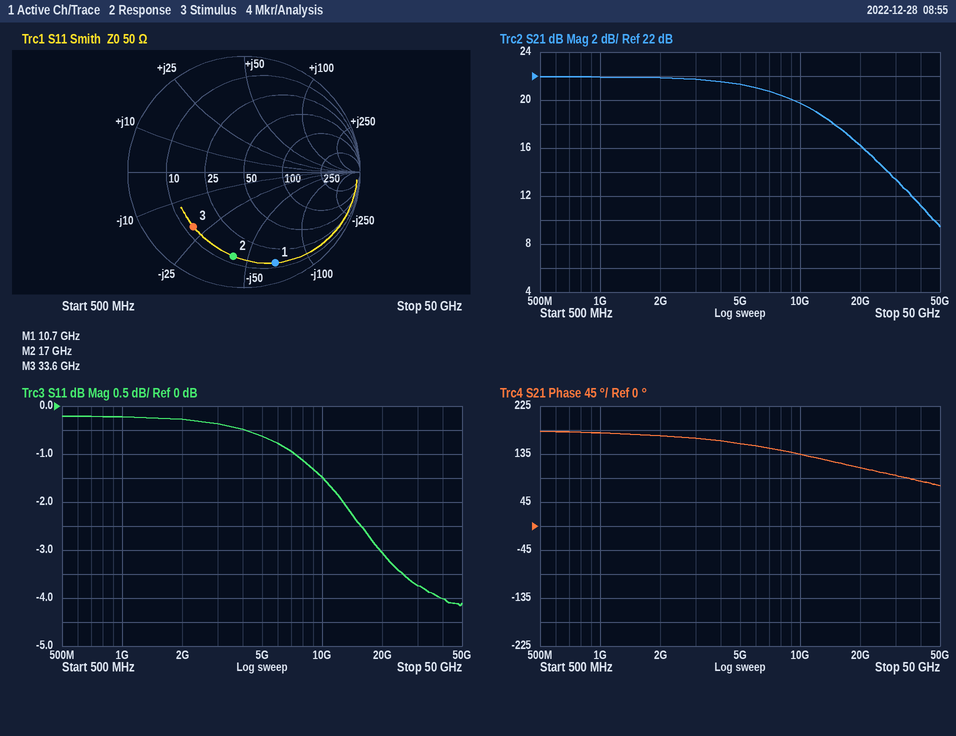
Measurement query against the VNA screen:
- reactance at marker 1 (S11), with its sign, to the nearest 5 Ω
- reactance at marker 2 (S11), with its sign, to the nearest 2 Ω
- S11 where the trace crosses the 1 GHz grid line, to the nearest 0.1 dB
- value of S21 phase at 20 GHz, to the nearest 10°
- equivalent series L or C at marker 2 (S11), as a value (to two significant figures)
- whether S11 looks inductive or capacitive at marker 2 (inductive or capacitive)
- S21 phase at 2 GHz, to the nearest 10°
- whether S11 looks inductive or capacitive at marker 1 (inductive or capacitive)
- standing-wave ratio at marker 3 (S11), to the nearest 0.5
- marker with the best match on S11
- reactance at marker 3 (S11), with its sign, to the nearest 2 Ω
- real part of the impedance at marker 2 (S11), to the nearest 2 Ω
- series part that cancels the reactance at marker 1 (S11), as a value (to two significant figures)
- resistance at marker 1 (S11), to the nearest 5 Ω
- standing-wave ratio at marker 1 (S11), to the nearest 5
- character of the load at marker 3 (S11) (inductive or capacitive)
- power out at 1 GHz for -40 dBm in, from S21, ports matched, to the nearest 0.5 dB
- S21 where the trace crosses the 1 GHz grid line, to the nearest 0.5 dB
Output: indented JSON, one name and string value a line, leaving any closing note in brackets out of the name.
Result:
{
  "reactance at marker 1 (S11), with its sign, to the nearest 5 Ω": "-70 Ω",
  "reactance at marker 2 (S11), with its sign, to the nearest 2 Ω": "-42 Ω",
  "S11 where the trace crosses the 1 GHz grid line, to the nearest 0.1 dB": "-0.2 dB",
  "value of S21 phase at 20 GHz, to the nearest 10°": "110°",
  "equivalent series L or C at marker 2 (S11), as a value": "220 fF",
  "whether S11 looks inductive or capacitive at marker 2": "capacitive",
  "S21 phase at 2 GHz, to the nearest 10°": "170°",
  "whether S11 looks inductive or capacitive at marker 1": "capacitive",
  "standing-wave ratio at marker 3 (S11), to the nearest 0.5": "4.5",
  "marker with the best match on S11": "marker 3",
  "reactance at marker 3 (S11), with its sign, to the nearest 2 Ω": "-20 Ω",
  "real part of the impedance at marker 2 (S11), to the nearest 2 Ω": "14 Ω",
  "series part that cancels the reactance at marker 1 (S11), as a value": "1.0 nH",
  "resistance at marker 1 (S11), to the nearest 5 Ω": "15 Ω",
  "standing-wave ratio at marker 1 (S11), to the nearest 5": "10",
  "character of the load at marker 3 (S11)": "capacitive",
  "power out at 1 GHz for -40 dBm in, from S21, ports matched, to the nearest 0.5 dB": "-18.0 dBm",
  "S21 where the trace crosses the 1 GHz grid line, to the nearest 0.5 dB": "22.0 dB"
}
